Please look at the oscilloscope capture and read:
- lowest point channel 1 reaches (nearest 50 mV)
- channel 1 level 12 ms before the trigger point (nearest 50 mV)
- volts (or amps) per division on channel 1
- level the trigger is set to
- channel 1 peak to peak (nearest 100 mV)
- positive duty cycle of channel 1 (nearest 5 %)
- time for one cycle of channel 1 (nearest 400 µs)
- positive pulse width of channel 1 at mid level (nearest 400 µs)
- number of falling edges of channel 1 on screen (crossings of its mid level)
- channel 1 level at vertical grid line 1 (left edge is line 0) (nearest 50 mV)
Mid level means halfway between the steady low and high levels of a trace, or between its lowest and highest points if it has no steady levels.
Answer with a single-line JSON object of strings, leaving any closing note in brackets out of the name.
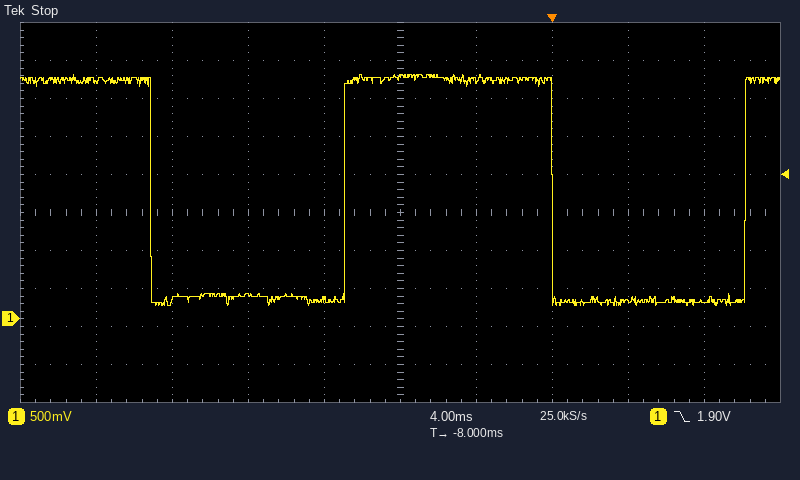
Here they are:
{"lowest point channel 1 reaches": "200 mV", "channel 1 level 12 ms before the trigger point": "250 mV", "volts (or amps) per division on channel 1": "500 mV", "level the trigger is set to": "1.90 V", "channel 1 peak to peak": "3.00 V", "positive duty cycle of channel 1": "50 %", "time for one cycle of channel 1": "21.2 ms", "positive pulse width of channel 1 at mid level": "10.8 ms", "number of falling edges of channel 1 on screen": "2", "channel 1 level at vertical grid line 1 (left edge is line 0)": "3.15 V"}
